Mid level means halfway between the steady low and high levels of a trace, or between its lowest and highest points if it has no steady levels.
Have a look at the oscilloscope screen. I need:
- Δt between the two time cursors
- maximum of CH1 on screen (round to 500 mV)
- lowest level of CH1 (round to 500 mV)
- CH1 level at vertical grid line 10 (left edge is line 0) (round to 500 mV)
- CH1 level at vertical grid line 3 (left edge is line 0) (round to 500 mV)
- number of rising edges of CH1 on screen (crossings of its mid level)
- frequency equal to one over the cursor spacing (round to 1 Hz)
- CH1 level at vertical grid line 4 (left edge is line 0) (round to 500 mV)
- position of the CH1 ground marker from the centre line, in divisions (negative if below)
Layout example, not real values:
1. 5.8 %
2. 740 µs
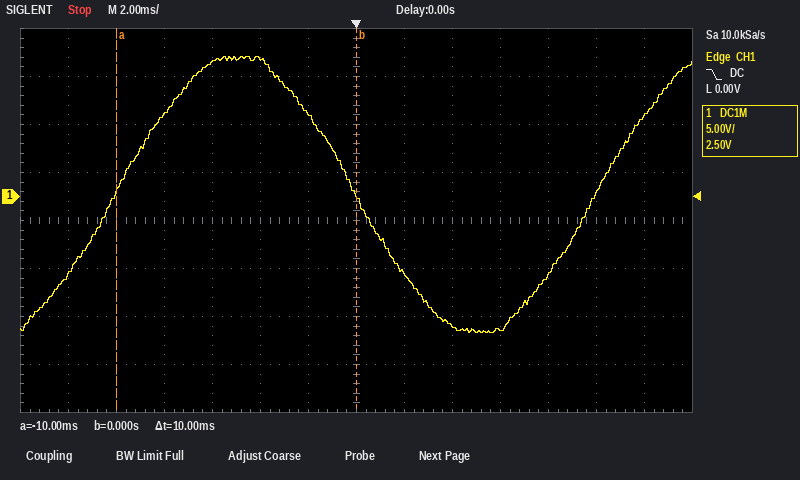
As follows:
1. 10 ms
2. 14.5 V
3. -14.0 V
4. -14.0 V
5. 8.5 V
6. 2
7. 100 Hz
8. 14.0 V
9. +0.5 div
